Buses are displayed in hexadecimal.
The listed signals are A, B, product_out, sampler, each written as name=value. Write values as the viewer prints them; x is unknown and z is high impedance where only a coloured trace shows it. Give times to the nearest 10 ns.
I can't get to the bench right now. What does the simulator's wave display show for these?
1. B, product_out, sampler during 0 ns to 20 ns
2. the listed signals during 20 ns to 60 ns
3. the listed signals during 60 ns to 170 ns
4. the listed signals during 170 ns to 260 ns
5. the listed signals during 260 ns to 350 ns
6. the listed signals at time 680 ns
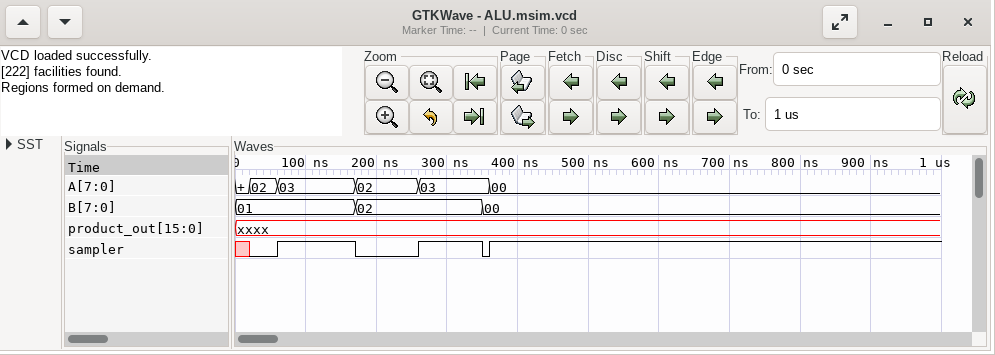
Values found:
B=01, product_out=xxxx, sampler=x
A=02, B=01, product_out=xxxx, sampler=0
A=03, B=01, product_out=xxxx, sampler=1
A=02, B=02, product_out=xxxx, sampler=0
A=03, B=02, product_out=xxxx, sampler=1
A=00, B=00, product_out=xxxx, sampler=1
